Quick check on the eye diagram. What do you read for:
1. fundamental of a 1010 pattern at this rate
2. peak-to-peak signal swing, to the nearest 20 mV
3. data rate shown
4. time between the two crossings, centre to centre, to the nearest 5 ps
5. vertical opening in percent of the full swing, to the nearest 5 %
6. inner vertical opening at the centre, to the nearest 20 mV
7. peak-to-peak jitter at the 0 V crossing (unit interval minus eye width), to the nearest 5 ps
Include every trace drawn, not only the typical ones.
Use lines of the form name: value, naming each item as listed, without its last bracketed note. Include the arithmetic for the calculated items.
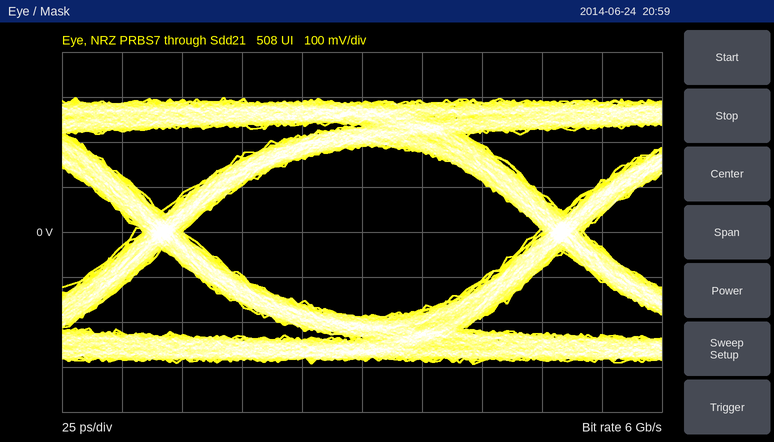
fundamental of a 1010 pattern at this rate: 3 GHz
peak-to-peak signal swing, to the nearest 20 mV: 600 mV
data rate shown: 6 Gb/s
time between the two crossings, centre to centre, to the nearest 5 ps: 165 ps
vertical opening in percent of the full swing, to the nearest 5 %: 380 mV / 600 mV ≈ 63.3 %, so 65 % to the nearest 5 %
inner vertical opening at the centre, to the nearest 20 mV: 380 mV
peak-to-peak jitter at the 0 V crossing (unit interval minus eye width), to the nearest 5 ps: 20 ps
